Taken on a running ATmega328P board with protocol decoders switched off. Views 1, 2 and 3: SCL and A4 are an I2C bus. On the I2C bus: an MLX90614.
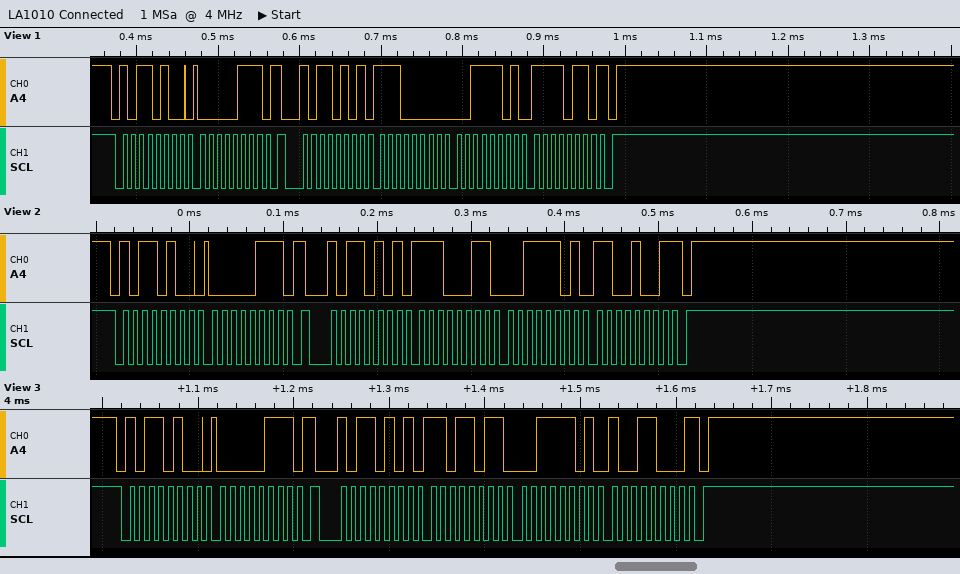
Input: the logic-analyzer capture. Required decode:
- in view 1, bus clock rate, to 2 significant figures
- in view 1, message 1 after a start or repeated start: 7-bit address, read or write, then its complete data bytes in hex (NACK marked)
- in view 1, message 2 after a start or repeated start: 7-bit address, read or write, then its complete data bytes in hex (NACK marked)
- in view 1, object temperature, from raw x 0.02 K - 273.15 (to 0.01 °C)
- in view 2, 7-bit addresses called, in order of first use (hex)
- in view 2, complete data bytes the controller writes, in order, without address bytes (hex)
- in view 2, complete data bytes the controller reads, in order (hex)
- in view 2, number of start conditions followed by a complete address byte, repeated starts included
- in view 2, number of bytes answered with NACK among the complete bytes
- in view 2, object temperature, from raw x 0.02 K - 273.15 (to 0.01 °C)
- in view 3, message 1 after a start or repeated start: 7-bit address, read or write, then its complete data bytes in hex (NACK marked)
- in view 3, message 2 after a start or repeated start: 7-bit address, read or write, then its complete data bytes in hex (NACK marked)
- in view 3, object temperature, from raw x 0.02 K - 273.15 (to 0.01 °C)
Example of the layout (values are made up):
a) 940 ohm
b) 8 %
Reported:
a) 100 kHz
b) 0x5A write: 07
c) 0x5A read: E0 3D F6 NACK
d) 43.65 °C
e) 0x5A
f) 07
g) E3 3D C9
h) 2
i) 1
j) 43.71 °C
k) 0x5A write: 07
l) 0x5A read: DB 3D 98 NACK
m) 43.55 °C
